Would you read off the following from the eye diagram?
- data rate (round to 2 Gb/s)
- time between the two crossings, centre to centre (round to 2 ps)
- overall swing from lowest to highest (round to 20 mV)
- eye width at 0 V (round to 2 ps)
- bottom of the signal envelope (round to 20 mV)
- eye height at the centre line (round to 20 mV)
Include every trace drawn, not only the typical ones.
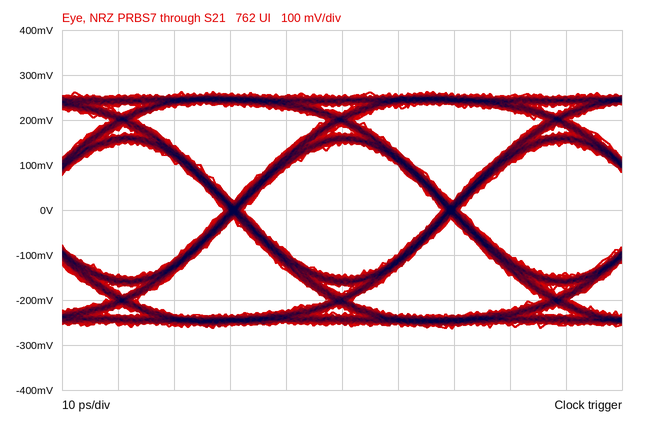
26 Gb/s
38 ps
520 mV
36 ps
-260 mV
300 mV
